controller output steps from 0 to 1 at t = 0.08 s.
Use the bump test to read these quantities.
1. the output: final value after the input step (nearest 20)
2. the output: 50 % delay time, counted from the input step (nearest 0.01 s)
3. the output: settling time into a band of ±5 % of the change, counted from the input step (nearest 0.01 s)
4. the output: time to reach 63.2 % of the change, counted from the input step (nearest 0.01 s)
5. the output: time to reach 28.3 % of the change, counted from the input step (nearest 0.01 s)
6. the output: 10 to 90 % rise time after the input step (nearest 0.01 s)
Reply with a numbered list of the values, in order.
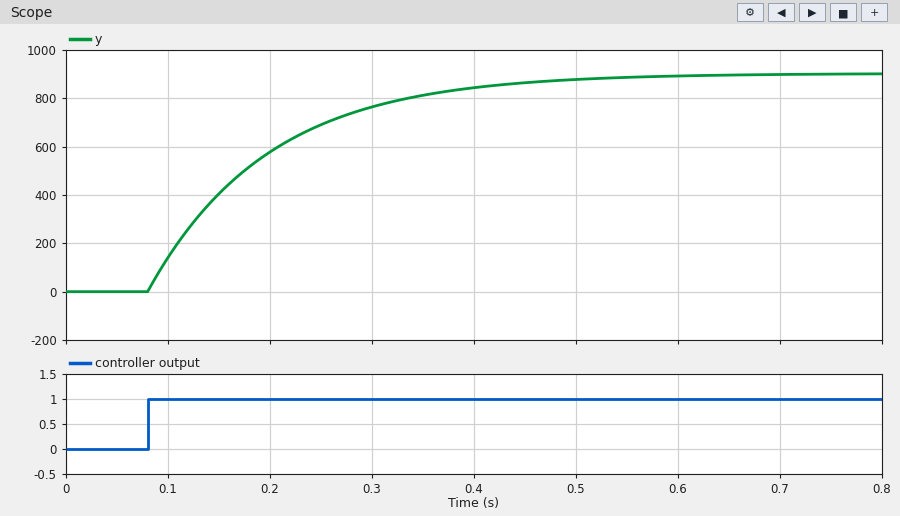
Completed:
1. 900
2. 0.08 s
3. 0.35 s
4. 0.12 s
5. 0.04 s
6. 0.26 s
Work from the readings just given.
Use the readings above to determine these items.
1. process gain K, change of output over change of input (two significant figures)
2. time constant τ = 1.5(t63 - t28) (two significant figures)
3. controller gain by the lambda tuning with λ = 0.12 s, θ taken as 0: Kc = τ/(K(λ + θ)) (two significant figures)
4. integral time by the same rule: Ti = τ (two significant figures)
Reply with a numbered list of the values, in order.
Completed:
1. 900
2. 0.12 s
3. 0.0011
4. 0.12 s
